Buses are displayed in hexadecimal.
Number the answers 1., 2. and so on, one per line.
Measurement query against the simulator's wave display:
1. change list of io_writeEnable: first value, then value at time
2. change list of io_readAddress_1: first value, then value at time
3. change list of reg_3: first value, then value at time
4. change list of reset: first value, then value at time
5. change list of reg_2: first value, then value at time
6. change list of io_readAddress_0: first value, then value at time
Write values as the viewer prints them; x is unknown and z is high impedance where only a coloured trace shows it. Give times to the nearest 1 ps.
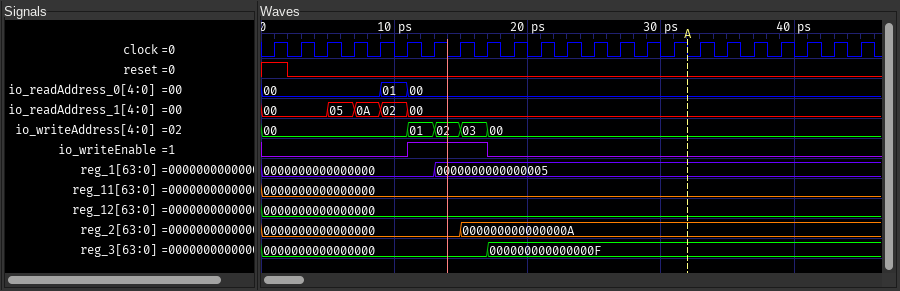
1. 0, 1 at 11 ps, 0 at 17 ps
2. 00, 05 at 5 ps, 0A at 7 ps, 02 at 9 ps, 00 at 11 ps
3. 0000000000000000, 000000000000000F at 17 ps
4. 1, 0 at 2 ps
5. 0000000000000000, 000000000000000A at 15 ps
6. 00, 01 at 9 ps, 00 at 11 ps
